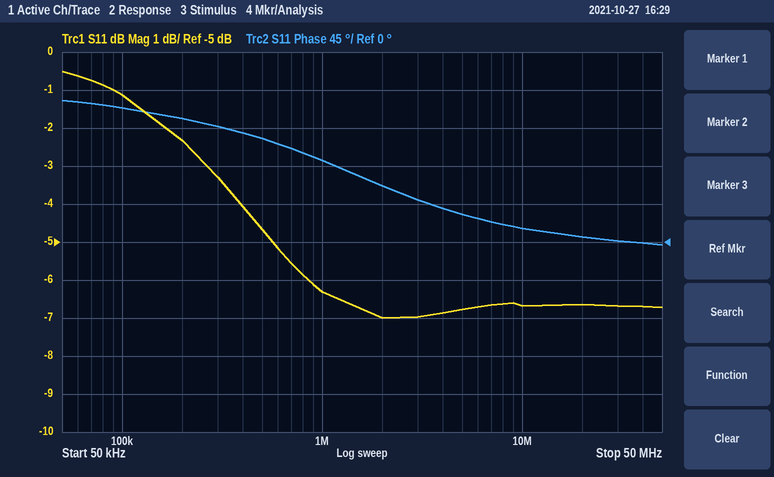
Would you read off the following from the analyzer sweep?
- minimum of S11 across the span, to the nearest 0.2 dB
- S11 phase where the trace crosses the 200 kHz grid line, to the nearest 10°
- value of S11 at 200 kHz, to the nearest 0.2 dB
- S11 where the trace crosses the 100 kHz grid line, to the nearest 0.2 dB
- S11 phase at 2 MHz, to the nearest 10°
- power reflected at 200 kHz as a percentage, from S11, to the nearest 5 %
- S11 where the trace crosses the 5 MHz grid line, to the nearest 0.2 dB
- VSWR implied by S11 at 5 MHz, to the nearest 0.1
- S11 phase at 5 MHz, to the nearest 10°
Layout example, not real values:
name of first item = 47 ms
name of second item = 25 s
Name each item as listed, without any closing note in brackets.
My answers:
minimum of S11 across the span, to the nearest 0.2 dB = -7.0 dB
S11 phase where the trace crosses the 200 kHz grid line, to the nearest 10° = 150°
value of S11 at 200 kHz, to the nearest 0.2 dB = -2.4 dB
S11 where the trace crosses the 100 kHz grid line, to the nearest 0.2 dB = -1.2 dB
S11 phase at 2 MHz, to the nearest 10° = 70°
power reflected at 200 kHz as a percentage, from S11, to the nearest 5 % = 60 %
S11 where the trace crosses the 5 MHz grid line, to the nearest 0.2 dB = -6.8 dB
VSWR implied by S11 at 5 MHz, to the nearest 0.1 = 2.7
S11 phase at 5 MHz, to the nearest 10° = 30°
